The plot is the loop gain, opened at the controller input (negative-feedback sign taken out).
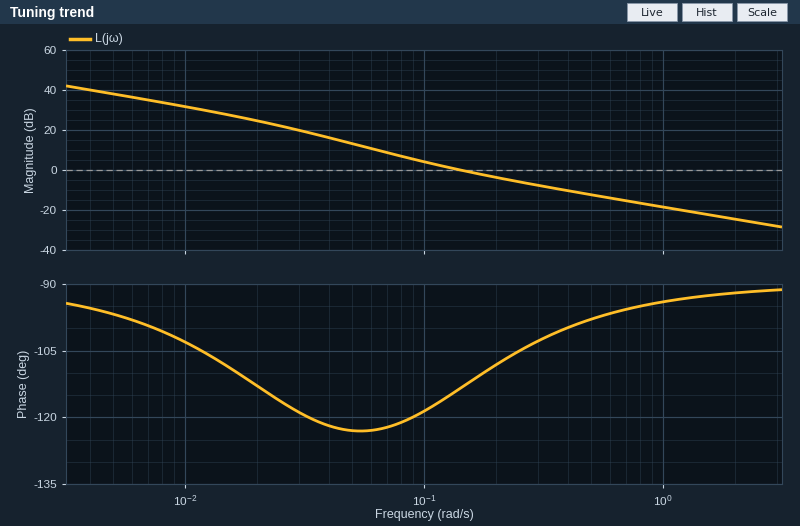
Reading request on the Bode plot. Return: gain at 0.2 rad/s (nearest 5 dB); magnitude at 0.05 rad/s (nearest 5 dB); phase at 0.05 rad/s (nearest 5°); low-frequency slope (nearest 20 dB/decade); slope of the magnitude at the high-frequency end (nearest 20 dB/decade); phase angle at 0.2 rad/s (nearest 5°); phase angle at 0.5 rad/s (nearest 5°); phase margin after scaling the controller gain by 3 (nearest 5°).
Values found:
-5 dB
15 dB
-125°
-20 dB/decade
-20 dB/decade
-110°
-100°
80°
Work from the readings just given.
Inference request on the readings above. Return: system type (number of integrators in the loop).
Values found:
1
